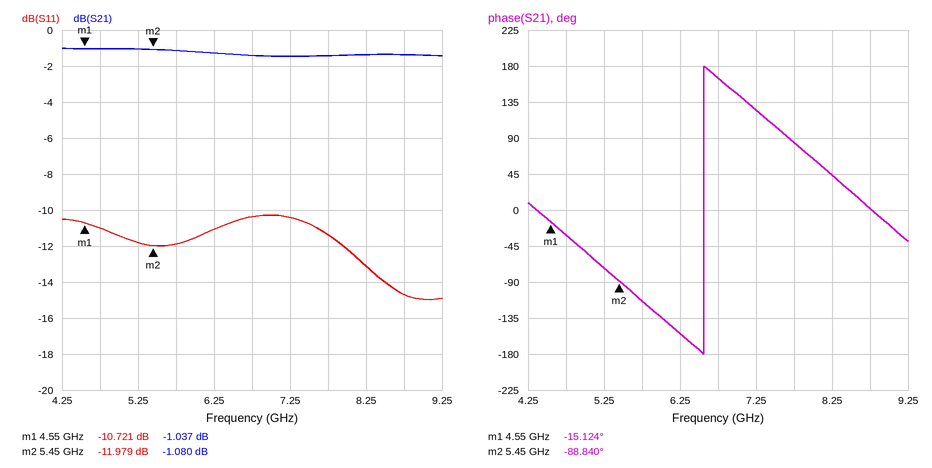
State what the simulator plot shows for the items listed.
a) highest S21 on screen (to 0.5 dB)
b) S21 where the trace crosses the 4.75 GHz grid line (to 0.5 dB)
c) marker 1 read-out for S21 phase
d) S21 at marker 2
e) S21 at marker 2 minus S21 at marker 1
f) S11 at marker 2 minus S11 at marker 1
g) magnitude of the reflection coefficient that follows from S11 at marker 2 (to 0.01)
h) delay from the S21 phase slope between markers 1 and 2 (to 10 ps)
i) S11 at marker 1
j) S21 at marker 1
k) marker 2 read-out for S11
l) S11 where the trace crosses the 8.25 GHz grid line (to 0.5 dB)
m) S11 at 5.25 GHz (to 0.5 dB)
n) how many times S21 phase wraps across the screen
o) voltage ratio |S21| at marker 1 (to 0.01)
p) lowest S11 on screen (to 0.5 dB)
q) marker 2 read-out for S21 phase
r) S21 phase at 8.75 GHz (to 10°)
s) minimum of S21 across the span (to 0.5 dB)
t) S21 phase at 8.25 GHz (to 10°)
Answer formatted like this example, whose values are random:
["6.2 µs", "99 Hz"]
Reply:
["-1.0 dB", "-1.0 dB", "-15.124°", "-1.080 dB", "-0.043 dB", "-1.258 dB", "0.25", "230 ps", "-10.721 dB", "-1.037 dB", "-11.979 dB", "-13.0 dB", "-12.0 dB", "1", "0.89", "-15.0 dB", "-88.840°", "0°", "-1.5 dB", "40°"]
